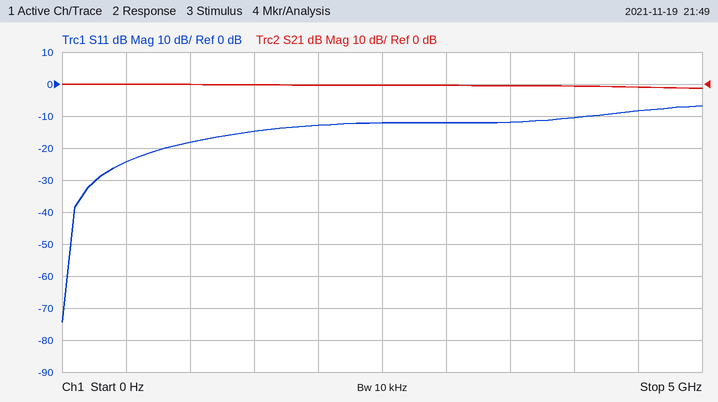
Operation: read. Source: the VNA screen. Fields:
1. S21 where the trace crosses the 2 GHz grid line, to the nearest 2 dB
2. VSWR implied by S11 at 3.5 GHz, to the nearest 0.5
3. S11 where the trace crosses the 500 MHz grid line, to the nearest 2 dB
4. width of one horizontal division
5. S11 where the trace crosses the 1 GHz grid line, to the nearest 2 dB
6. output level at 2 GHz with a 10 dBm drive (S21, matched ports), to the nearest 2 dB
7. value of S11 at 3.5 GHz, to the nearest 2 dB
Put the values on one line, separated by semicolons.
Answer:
0 dB; 1.5; -24 dB; 500 MHz; -18 dB; 10 dBm; -12 dB
